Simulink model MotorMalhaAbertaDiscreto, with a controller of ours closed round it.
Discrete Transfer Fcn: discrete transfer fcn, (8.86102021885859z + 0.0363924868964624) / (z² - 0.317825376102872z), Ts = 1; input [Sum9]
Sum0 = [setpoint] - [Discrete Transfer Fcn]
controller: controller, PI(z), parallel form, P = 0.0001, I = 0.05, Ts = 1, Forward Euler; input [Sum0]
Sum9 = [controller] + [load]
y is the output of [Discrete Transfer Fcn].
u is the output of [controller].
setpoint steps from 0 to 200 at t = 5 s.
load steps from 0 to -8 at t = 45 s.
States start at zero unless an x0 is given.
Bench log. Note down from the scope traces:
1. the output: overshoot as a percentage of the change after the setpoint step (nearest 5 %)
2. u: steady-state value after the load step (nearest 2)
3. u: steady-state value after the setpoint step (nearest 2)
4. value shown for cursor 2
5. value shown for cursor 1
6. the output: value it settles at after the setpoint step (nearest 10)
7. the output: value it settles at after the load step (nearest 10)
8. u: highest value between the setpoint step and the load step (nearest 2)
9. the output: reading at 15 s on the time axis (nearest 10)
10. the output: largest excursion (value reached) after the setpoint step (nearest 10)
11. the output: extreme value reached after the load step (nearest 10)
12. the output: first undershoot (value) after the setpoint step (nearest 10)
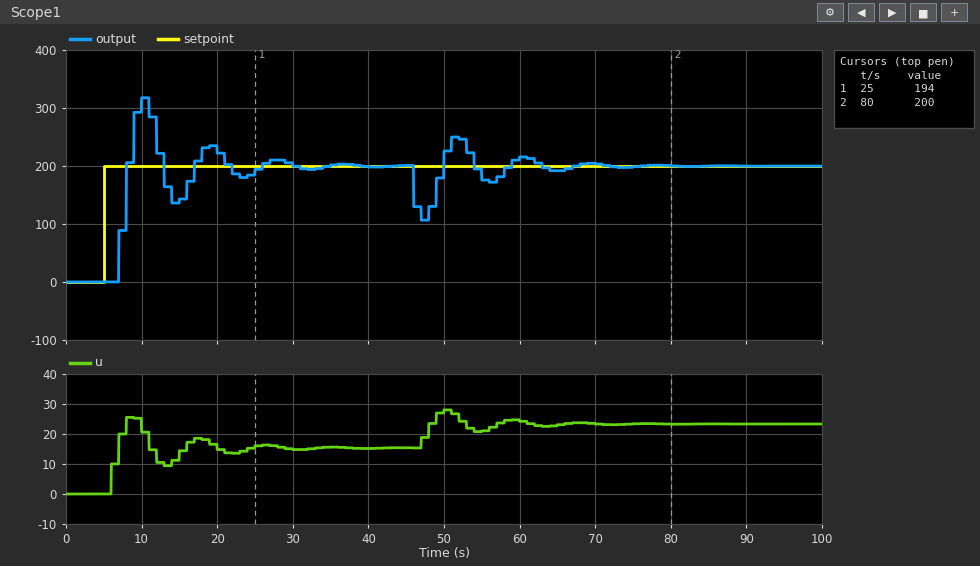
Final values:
60 %
24
16
200
194
200
200
26
140
320
110
140
